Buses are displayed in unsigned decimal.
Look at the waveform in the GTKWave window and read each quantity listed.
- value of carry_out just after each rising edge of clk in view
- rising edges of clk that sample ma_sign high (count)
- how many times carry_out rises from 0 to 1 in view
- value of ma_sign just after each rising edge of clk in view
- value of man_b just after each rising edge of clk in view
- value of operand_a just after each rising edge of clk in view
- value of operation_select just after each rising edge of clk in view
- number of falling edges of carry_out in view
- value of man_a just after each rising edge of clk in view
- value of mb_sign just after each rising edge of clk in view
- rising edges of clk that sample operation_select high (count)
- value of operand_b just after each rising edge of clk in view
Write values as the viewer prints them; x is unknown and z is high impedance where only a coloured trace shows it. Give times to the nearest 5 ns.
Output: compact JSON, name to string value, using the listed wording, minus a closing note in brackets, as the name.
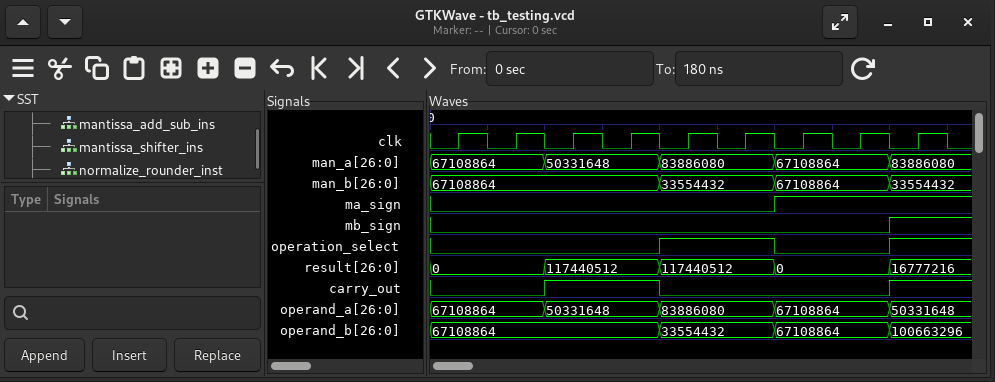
{"value of carry_out just after each rising edge of clk in view": "0 0 1 1 0 0 0 0 1", "rising edges of clk that sample ma_sign high": "3", "how many times carry_out rises from 0 to 1 in view": "2", "value of ma_sign just after each rising edge of clk in view": "0 0 0 0 0 0 1 1 1", "value of man_b just after each rising edge of clk in view": "67108864, 67108864, 67108864, 67108864, 33554432, 33554432, 67108864, 67108864, 33554432", "value of operand_a just after each rising edge of clk in view": "67108864, 67108864, 50331648, 50331648, 83886080, 83886080, 67108864, 67108864, 50331648", "value of operation_select just after each rising edge of clk in view": "0 0 0 0 1 1 0 0 1", "number of falling edges of carry_out in view": "1", "value of man_a just after each rising edge of clk in view": "67108864, 67108864, 50331648, 50331648, 83886080, 83886080, 67108864, 67108864, 83886080", "value of mb_sign just after each rising edge of clk in view": "0 0 0 0 0 0 0 0 1", "rising edges of clk that sample operation_select high": "3", "value of operand_b just after each rising edge of clk in view": "67108864, 67108864, 67108864, 67108864, 33554432, 33554432, 67108864, 67108864, 100663296"}
